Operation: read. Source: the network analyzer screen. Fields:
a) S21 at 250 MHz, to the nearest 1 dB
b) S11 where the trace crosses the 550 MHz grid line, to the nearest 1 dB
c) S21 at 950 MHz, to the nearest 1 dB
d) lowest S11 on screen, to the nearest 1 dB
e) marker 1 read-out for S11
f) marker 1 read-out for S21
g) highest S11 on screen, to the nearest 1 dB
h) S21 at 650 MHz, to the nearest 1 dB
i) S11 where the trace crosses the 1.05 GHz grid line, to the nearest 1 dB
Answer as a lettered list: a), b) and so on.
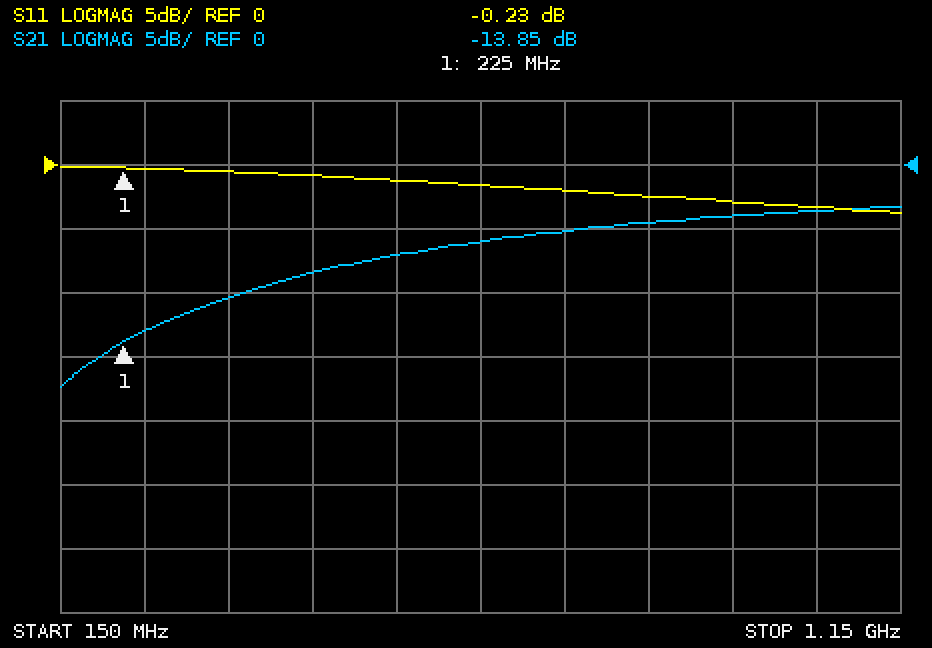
a) -13 dB
b) -1 dB
c) -4 dB
d) -4 dB
e) -0.23 dB
f) -13.85 dB
g) 0 dB
h) -6 dB
i) -3 dB
